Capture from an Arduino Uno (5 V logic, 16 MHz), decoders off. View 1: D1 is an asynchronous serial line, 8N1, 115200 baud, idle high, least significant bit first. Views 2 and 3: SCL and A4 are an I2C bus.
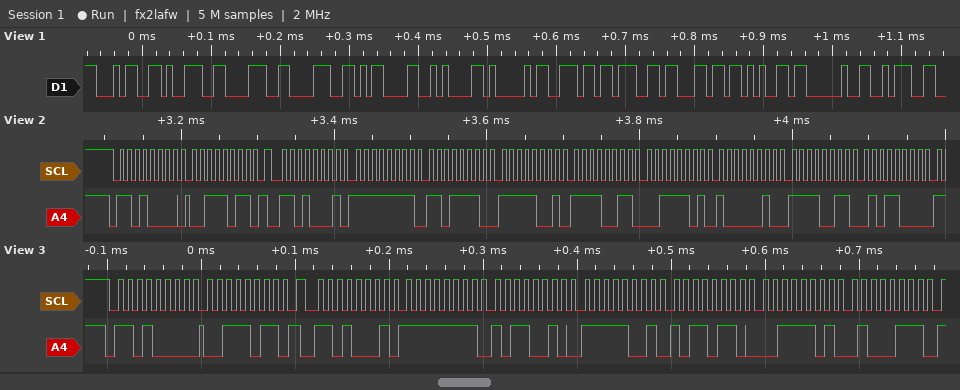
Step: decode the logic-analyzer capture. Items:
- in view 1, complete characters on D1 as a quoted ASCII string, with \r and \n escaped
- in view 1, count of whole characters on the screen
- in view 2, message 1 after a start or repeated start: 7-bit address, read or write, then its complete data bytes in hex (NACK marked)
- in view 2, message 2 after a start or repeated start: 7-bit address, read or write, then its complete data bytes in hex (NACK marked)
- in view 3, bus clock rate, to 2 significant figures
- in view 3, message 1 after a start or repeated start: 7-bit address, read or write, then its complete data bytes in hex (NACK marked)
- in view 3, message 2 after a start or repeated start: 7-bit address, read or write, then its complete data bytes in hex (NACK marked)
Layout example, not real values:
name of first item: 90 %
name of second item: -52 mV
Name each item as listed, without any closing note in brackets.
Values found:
in view 1, complete characters on D1 as a quoted ASCII string, with \r and \n escaped: "4988\r\nAngle :"
in view 1, count of whole characters on the screen: 13
in view 2, message 1 after a start or repeated start: 7-bit address, read or write, then its complete data bytes in hex: 0x68 write: 3B
in view 2, message 2 after a start or repeated start: 7-bit address, read or write, then its complete data bytes in hex: 0x68 read: FF DE F9 F3 3D 82 F3 58
in view 3, bus clock rate, to 2 significant figures: 100 kHz
in view 3, message 1 after a start or repeated start: 7-bit address, read or write, then its complete data bytes in hex: 0x68 write: 3B
in view 3, message 2 after a start or repeated start: 7-bit address, read or write, then its complete data bytes in hex: 0x68 read: FF B2 F9 B6 3D 47
